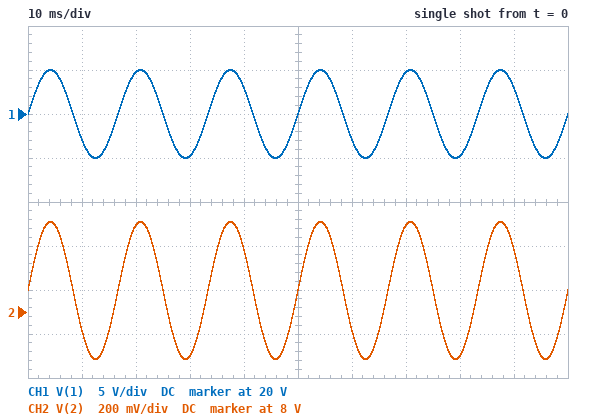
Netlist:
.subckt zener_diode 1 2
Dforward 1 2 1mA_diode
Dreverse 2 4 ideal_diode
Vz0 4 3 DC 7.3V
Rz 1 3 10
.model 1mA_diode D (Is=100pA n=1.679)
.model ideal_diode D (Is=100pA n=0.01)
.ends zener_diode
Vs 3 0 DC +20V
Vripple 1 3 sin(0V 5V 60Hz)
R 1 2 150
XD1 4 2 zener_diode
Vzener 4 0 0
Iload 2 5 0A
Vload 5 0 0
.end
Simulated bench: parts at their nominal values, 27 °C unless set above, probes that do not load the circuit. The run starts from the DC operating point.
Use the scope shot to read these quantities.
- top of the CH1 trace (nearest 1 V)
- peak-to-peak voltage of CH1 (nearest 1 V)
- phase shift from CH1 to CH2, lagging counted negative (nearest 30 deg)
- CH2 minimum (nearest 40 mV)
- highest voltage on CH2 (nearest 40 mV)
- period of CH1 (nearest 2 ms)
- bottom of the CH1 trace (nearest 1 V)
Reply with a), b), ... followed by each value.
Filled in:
a) 25 V
b) 10 V
c) 0 deg
d) 7.80 V
e) 8.40 V
f) 16 ms
g) 15 V
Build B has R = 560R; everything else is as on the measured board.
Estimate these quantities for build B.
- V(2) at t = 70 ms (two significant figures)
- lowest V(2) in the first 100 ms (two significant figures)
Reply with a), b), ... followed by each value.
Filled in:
a) 7.6 V
b) 7.4 V
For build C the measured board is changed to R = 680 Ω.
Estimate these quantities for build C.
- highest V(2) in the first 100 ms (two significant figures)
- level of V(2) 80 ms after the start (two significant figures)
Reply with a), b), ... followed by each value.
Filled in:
a) 7.6 V
b) 7.4 V
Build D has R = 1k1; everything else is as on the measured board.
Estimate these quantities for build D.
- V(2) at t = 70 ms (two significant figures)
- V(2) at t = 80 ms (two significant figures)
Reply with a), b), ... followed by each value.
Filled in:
a) 7.5 V
b) 7.4 V
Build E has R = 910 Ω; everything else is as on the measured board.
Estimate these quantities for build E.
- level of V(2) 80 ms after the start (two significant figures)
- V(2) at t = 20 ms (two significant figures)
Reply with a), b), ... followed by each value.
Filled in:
a) 7.4 V
b) 7.5 V
